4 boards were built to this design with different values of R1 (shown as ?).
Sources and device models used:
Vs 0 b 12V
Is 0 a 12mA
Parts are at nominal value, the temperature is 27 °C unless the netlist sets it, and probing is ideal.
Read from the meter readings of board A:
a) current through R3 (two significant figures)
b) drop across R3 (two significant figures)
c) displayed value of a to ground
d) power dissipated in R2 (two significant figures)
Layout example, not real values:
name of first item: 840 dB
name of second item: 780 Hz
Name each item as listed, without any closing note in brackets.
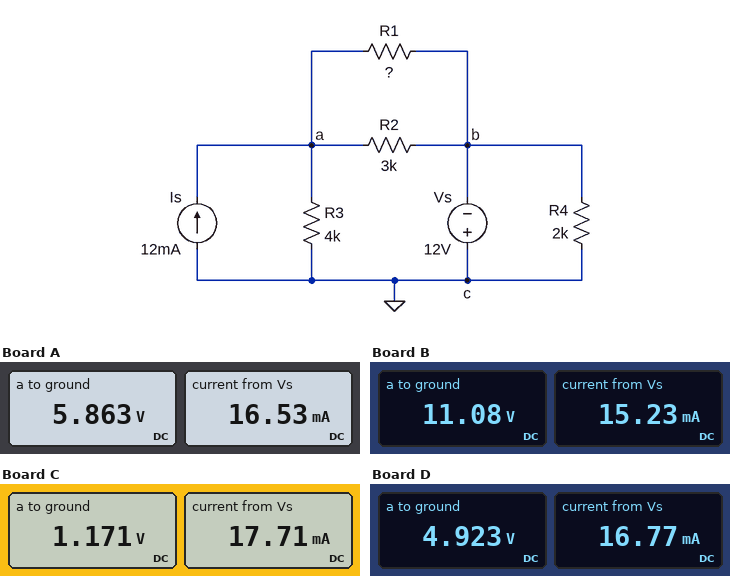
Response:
current through R3: 1.5 mA
drop across R3: 5.9 V
displayed value of a to ground: 5.863 V
power dissipated in R2: 110 mW
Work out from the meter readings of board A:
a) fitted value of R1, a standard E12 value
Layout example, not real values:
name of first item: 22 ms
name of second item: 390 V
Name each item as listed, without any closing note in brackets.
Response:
fitted value of R1, a standard E12 value: 3.9 kΩ
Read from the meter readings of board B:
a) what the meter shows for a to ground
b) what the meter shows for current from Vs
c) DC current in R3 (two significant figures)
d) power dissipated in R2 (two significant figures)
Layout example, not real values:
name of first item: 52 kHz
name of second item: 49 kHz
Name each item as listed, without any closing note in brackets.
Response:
what the meter shows for a to ground: 11.08 V
what the meter shows for current from Vs: 15.23 mA
DC current in R3: 2.8 mA
power dissipated in R2: 180 mW
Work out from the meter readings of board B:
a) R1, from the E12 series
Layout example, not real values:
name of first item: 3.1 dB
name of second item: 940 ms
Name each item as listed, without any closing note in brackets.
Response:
R1, from the E12 series: 15 kΩ
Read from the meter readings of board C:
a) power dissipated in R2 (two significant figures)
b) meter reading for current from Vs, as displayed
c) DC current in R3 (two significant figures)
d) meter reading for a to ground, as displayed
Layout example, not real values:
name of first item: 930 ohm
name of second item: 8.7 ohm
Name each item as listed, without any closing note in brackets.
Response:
power dissipated in R2: 58 mW
meter reading for current from Vs, as displayed: 17.71 mA
DC current in R3: 290 µA
meter reading for a to ground, as displayed: 1.171 V
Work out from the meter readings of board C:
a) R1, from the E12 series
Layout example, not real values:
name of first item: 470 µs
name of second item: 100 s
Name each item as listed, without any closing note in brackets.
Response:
R1, from the E12 series: 1.8 kΩ
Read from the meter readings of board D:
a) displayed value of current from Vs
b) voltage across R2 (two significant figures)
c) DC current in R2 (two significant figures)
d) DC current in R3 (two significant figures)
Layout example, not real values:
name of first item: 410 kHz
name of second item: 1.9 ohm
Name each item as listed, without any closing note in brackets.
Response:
displayed value of current from Vs: 16.77 mA
voltage across R2: 17 V
DC current in R2: 5.6 mA
DC current in R3: 1.2 mA
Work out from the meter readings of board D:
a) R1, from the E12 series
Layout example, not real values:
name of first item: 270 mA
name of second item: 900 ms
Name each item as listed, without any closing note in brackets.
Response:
R1, from the E12 series: 3.3 kΩ
